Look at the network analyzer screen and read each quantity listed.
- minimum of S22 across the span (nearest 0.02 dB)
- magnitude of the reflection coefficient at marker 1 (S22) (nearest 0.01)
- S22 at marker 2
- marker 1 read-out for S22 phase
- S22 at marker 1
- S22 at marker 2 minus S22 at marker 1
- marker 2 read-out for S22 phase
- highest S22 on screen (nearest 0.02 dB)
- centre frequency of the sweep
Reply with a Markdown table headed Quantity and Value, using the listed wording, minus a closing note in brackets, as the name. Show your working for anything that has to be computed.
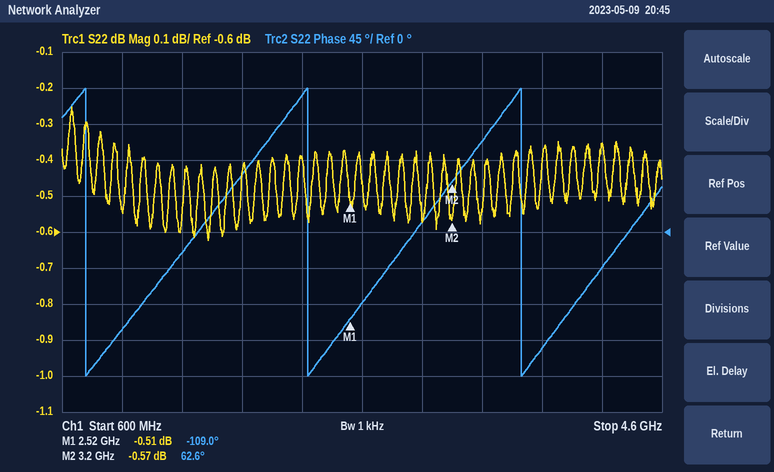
| Quantity | Value |
|---|---|
| minimum of S22 across the span | -0.62 dB |
| magnitude of the reflection coefficient at marker 1 (S22) | 10^(-0.51/20) ≈ 0.94 |
| S22 at marker 2 | -0.57 dB |
| marker 1 read-out for S22 phase | -109.0° |
| S22 at marker 1 | -0.51 dB |
| S22 at marker 2 minus S22 at marker 1 | -0.57 − (-0.51) = -0.06 dB |
| marker 2 read-out for S22 phase | 62.6° |
| highest S22 on screen | -0.26 dB |
| centre frequency of the sweep | 2.6 GHz |
